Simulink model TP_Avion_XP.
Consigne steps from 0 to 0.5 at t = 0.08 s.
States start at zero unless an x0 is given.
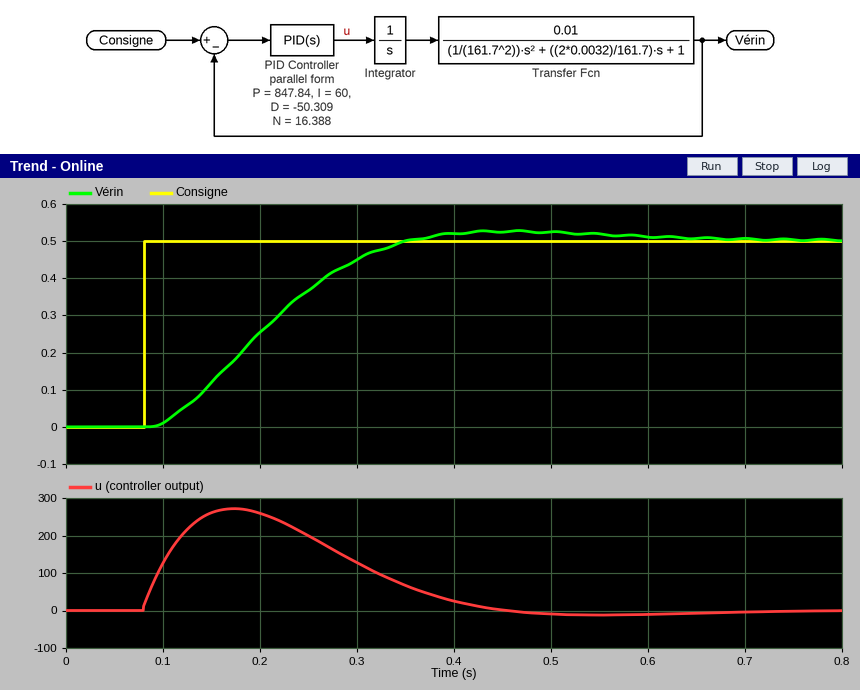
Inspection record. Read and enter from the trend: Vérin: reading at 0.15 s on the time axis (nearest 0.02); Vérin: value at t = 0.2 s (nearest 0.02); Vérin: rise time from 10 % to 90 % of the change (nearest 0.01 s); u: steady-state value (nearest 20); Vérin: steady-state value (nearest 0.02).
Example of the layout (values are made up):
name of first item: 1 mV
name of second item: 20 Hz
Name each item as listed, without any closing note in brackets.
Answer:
Vérin: reading at 0.15 s on the time axis: 0.12
Vérin: value at t = 0.2 s: 0.26
Vérin: rise time from 10 % to 90 % of the change: 0.18 s
u: steady-state value: 0
Vérin: steady-state value: 0.50
